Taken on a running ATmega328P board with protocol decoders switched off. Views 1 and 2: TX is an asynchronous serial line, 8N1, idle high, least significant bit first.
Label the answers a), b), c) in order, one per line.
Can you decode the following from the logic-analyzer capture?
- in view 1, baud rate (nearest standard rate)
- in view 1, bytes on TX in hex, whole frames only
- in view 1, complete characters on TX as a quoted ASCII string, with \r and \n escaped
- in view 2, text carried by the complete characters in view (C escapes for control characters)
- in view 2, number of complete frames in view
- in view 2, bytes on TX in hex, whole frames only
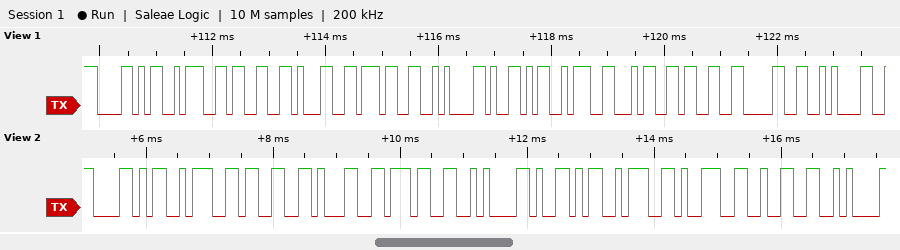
a) 9600 baud
b) 58 3A 33 31 37 0A 59 3A 34 33 30 0A
c) "X:317\nY:430\n"
d) "X:317\nY:92\n"
e) 11
f) 58 3A 33 31 37 0A 59 3A 39 32 0A
